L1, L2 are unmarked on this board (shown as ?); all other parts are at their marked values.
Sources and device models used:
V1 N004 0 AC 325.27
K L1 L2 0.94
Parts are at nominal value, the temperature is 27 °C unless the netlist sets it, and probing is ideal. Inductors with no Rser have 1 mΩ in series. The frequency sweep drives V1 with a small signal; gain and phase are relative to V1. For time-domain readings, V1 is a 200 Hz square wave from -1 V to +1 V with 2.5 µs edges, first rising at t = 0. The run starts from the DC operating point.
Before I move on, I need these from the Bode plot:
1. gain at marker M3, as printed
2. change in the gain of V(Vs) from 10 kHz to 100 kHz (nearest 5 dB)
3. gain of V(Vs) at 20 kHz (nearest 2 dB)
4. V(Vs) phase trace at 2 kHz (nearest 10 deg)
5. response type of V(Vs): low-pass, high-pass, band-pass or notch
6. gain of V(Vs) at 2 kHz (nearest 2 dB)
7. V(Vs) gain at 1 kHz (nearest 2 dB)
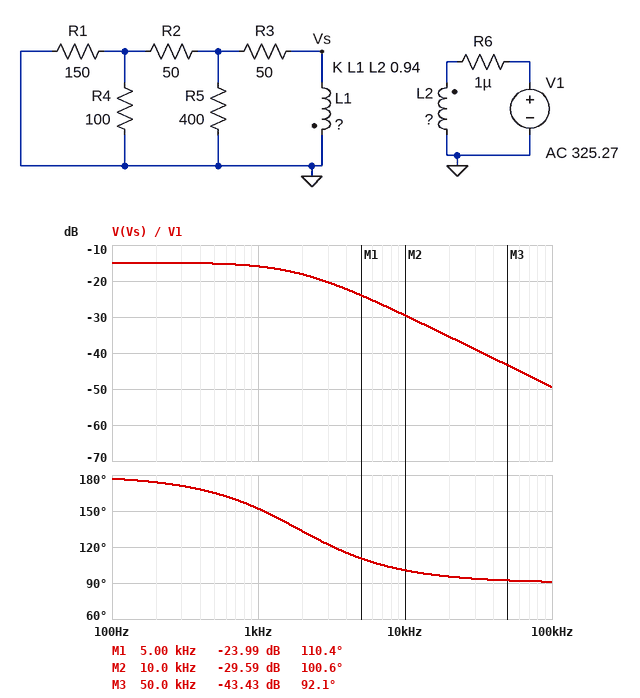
-43.43 dB
-20 dB
-36 dB
130 deg
low-pass
-18 dB
-16 dB
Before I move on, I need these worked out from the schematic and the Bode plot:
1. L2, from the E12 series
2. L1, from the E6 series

2.7 H
100 mH
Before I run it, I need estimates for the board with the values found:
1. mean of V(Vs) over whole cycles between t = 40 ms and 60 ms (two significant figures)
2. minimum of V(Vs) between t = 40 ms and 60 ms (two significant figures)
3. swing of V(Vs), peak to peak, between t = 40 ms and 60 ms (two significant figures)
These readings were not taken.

-180 mV
-360 mV
360 mV
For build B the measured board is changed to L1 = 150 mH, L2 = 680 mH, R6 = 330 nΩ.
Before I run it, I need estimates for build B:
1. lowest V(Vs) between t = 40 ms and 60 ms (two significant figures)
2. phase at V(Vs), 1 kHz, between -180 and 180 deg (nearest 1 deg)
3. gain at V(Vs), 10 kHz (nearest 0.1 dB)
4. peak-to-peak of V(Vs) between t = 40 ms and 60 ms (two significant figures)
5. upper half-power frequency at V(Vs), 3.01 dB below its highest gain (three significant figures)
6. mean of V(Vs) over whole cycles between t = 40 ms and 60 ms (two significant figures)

-880 mV
141 deg
-25.3 dB
880 mV
1.24 kHz
-440 mV
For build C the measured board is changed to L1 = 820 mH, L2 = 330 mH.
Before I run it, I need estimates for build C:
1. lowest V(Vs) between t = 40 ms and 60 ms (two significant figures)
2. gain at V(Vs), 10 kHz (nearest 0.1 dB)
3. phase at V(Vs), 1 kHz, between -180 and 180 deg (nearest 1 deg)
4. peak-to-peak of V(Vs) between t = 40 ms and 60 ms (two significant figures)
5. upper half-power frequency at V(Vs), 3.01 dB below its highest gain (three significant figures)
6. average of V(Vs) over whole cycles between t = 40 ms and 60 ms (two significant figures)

-2.9 V
-29.5 dB
103 deg
2.8 V
227 Hz
-1.5 V
